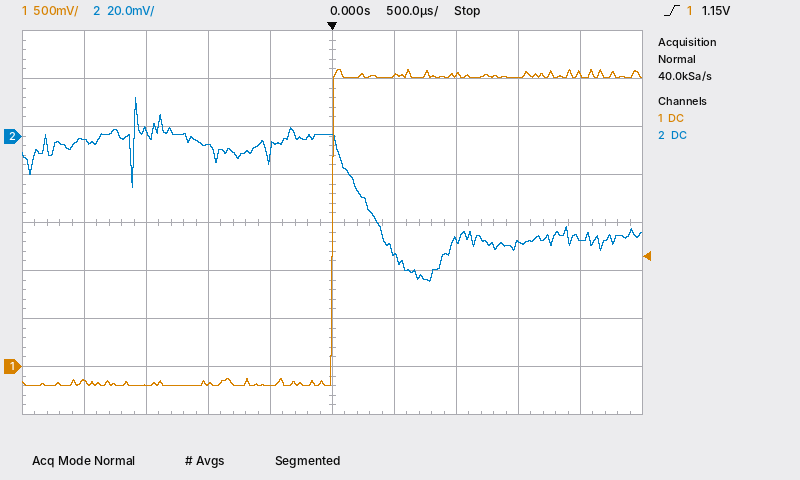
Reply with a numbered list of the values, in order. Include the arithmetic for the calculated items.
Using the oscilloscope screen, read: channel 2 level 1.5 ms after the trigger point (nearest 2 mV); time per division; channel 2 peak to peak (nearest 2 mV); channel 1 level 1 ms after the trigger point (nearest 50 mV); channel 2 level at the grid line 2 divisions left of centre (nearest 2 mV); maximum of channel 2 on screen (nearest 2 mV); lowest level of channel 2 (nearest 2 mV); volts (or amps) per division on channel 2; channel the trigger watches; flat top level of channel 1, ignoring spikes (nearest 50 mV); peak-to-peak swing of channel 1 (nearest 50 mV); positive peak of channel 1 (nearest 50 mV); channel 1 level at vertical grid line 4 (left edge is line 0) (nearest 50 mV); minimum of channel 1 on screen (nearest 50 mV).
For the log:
1. -44 mV
2. 500 µs
3. 16 mV − (-60 mV) = 76 mV
4. 3.05 V
5. -4 mV
6. 16 mV
7. -60 mV
8. 20 mV
9. channel 1
10. 3.00 V
11. 3.10 V − (-200 mV) = 3.30 V
12. 3.10 V
13. -200 mV
14. -200 mV
